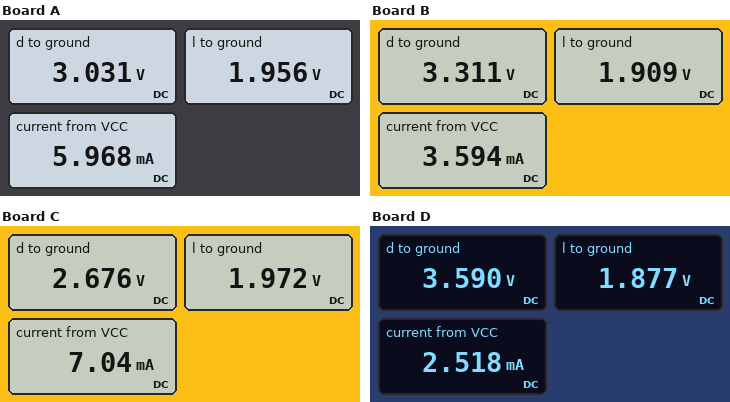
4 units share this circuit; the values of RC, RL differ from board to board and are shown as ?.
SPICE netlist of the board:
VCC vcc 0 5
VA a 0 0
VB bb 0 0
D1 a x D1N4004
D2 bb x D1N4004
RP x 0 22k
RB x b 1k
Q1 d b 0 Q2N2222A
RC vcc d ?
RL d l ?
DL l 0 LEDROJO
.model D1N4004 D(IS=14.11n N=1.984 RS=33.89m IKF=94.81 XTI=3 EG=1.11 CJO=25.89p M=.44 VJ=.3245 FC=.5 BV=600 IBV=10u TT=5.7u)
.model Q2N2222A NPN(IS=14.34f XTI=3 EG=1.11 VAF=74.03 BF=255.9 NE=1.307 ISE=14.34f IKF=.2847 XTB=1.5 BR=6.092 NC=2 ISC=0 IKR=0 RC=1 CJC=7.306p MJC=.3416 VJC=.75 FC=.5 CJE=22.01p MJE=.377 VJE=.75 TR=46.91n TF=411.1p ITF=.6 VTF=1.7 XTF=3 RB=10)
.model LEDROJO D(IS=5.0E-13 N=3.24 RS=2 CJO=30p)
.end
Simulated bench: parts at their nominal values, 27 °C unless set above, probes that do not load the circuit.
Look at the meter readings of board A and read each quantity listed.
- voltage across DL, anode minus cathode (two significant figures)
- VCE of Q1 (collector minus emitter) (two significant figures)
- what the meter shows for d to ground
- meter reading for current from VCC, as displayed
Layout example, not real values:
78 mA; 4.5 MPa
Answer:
2.0 V; 3.0 V; 3.031 V; 5.968 mA
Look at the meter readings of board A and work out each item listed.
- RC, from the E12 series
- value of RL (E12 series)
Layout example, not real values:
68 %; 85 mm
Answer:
330 Ω; 180 Ω
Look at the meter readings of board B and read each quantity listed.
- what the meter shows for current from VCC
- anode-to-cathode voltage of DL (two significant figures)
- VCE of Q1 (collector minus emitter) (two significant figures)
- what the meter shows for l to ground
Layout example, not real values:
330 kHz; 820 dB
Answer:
3.594 mA; 1.9 V; 3.3 V; 1.909 V
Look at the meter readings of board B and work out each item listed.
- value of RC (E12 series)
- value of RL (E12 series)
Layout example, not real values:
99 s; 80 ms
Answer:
470 Ω; 390 Ω
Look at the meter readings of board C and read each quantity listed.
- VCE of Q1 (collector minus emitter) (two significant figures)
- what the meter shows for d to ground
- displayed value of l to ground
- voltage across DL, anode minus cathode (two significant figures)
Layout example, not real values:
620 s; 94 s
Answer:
2.7 V; 2.676 V; 1.972 V; 2.0 V
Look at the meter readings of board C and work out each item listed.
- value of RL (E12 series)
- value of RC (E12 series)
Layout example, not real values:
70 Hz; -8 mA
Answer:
100 Ω; 330 Ω
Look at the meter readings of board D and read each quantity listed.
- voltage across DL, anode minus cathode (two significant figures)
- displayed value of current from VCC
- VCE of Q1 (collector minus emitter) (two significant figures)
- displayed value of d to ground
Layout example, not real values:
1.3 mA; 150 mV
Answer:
1.9 V; 2.518 mA; 3.6 V; 3.590 V
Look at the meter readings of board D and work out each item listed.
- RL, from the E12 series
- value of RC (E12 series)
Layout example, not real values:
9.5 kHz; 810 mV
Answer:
680 Ω; 560 Ω
